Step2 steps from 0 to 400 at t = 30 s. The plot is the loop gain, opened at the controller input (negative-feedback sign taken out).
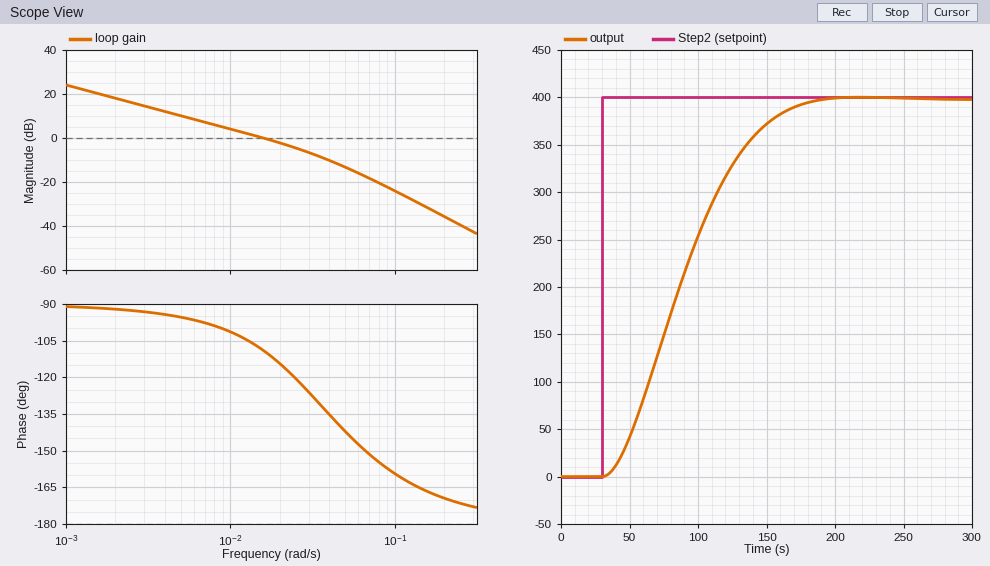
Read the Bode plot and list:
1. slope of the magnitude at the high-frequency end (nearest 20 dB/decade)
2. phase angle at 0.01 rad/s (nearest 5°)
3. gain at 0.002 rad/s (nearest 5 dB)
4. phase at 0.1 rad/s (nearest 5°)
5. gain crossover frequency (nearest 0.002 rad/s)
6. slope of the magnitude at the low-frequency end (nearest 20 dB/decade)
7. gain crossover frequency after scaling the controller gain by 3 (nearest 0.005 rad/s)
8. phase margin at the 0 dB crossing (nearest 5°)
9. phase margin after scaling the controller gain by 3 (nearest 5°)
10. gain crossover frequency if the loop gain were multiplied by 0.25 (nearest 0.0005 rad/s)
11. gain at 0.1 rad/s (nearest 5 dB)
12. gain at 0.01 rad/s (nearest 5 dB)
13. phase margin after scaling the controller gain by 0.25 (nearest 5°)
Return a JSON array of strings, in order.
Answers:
["-40 dB/decade", "-100°", "20 dB", "-160°", "0.016 rad/s", "-20 dB/decade", "0.040 rad/s", "70°", "45°", "0.0040 rad/s", "-25 dB", "5 dB", "85°"]
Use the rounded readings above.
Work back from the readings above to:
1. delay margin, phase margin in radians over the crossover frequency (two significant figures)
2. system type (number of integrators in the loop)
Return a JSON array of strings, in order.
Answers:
["76 s", "1"]
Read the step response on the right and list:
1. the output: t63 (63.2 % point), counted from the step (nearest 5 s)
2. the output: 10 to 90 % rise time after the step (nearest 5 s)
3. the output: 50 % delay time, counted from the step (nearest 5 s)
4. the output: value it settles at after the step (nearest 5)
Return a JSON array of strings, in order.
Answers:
["70 s", "90 s", "55 s", "400"]
